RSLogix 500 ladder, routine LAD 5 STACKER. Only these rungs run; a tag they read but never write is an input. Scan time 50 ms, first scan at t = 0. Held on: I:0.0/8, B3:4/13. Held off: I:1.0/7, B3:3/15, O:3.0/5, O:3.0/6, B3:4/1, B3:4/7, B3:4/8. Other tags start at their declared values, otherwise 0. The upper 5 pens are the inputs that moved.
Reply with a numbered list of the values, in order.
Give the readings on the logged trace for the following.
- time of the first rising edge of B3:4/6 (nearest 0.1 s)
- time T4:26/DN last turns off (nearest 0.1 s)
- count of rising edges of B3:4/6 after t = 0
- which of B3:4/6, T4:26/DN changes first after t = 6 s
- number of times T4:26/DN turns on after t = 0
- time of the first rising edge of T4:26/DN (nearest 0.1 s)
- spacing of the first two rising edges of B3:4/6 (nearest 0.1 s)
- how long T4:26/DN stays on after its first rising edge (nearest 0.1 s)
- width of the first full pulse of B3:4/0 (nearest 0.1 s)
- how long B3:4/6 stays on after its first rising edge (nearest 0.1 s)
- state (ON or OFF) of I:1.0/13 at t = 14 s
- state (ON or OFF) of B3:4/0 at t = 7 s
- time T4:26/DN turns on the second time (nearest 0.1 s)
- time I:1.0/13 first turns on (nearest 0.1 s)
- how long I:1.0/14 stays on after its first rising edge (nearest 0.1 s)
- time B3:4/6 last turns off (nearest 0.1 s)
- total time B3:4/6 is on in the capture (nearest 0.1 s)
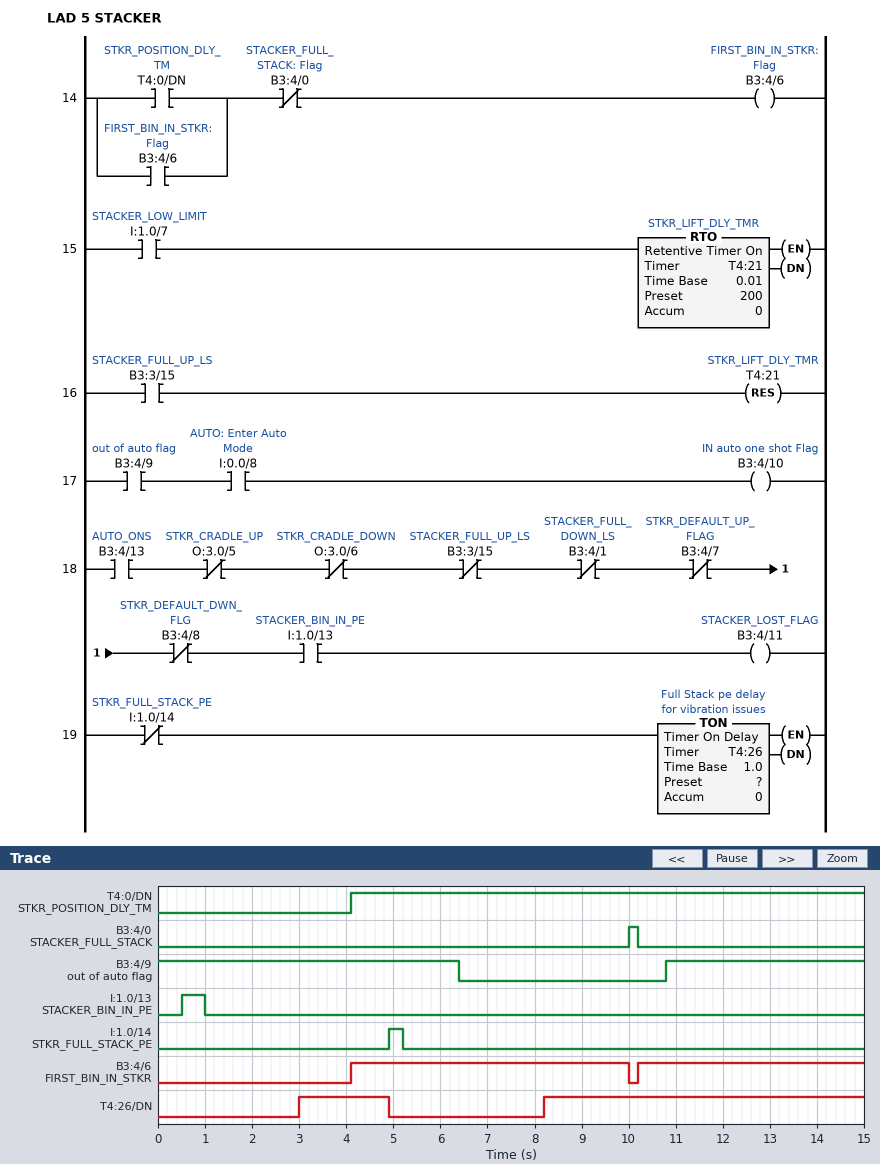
1. 4.1 s
2. 4.9 s
3. 2
4. T4:26/DN
5. 2
6. 3.0 s
7. 6.1 s
8. 1.9 s
9. 0.2 s
10. 5.9 s
11. OFF
12. OFF
13. 8.2 s
14. 0.5 s
15. 0.3 s
16. 10.0 s
17. 10.7 s
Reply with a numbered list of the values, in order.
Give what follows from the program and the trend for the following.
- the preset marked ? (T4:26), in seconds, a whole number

1. 3 s
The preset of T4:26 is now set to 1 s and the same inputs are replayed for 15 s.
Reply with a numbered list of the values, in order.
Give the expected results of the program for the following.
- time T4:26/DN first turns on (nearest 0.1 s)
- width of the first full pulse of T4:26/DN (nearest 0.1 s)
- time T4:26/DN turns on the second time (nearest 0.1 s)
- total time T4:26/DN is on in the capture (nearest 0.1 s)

1. 1.0 s
2. 3.9 s
3. 6.2 s
4. 12.7 s
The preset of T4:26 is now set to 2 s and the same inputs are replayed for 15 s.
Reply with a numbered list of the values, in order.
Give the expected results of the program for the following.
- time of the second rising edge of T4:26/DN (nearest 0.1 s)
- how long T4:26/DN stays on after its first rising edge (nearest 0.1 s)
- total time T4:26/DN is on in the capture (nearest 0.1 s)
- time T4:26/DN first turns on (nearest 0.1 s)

1. 7.2 s
2. 2.9 s
3. 10.7 s
4. 2.0 s
